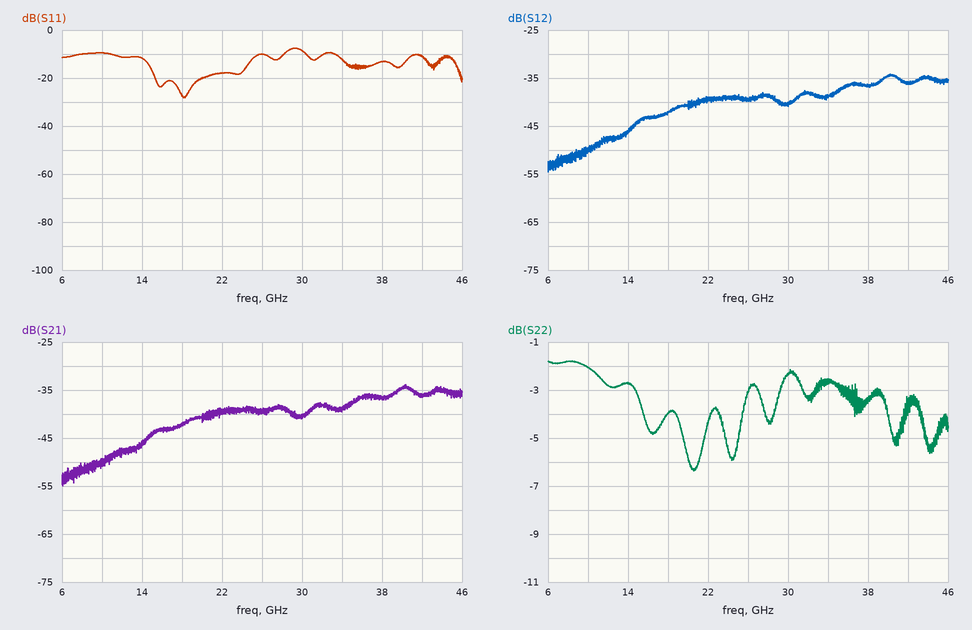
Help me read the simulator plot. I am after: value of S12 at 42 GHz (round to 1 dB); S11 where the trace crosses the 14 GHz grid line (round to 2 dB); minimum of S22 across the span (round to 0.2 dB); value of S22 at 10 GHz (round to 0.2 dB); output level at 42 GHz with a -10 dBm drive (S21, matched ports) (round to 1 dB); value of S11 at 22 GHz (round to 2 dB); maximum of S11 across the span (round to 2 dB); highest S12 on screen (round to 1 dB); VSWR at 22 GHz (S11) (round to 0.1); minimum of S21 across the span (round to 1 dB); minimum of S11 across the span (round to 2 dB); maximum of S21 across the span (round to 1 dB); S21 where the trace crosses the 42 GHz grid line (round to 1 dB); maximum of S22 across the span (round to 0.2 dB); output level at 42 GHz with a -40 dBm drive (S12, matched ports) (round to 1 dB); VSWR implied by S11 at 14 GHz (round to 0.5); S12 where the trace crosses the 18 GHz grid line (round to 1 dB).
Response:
-36 dB
-12 dB
-6.4 dB
-2.0 dB
-46 dBm
-18 dB
-8 dB
-34 dB
1.3
-55 dB
-28 dB
-34 dB
-36 dB
-1.8 dB
-76 dBm
1.5
-42 dB
